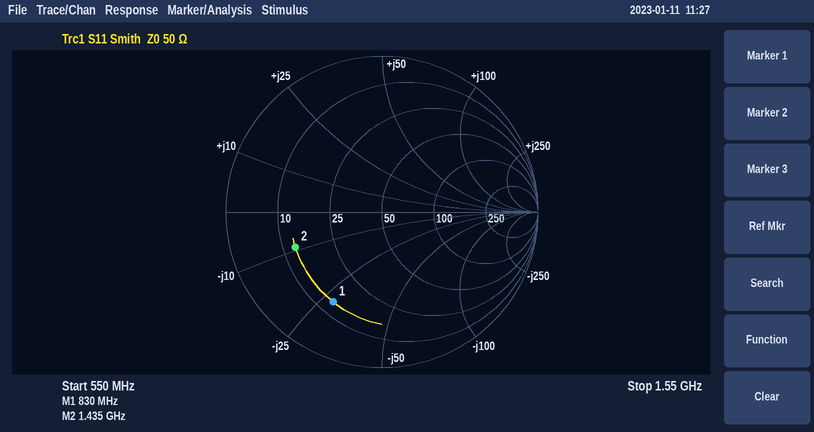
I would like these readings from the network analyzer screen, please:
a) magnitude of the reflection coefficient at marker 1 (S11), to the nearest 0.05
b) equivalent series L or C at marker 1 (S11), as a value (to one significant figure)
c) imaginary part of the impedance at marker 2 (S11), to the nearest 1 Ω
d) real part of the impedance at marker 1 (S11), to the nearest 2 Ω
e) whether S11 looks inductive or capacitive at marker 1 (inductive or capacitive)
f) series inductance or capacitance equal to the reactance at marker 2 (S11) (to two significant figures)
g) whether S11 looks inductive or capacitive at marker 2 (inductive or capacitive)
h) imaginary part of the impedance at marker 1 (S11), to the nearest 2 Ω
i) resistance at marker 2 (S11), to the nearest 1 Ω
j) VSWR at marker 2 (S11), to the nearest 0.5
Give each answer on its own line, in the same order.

0.65
7 pF
-9 Ω
14 Ω
capacitive
12 pF
capacitive
-28 Ω
13 Ω
4.0
